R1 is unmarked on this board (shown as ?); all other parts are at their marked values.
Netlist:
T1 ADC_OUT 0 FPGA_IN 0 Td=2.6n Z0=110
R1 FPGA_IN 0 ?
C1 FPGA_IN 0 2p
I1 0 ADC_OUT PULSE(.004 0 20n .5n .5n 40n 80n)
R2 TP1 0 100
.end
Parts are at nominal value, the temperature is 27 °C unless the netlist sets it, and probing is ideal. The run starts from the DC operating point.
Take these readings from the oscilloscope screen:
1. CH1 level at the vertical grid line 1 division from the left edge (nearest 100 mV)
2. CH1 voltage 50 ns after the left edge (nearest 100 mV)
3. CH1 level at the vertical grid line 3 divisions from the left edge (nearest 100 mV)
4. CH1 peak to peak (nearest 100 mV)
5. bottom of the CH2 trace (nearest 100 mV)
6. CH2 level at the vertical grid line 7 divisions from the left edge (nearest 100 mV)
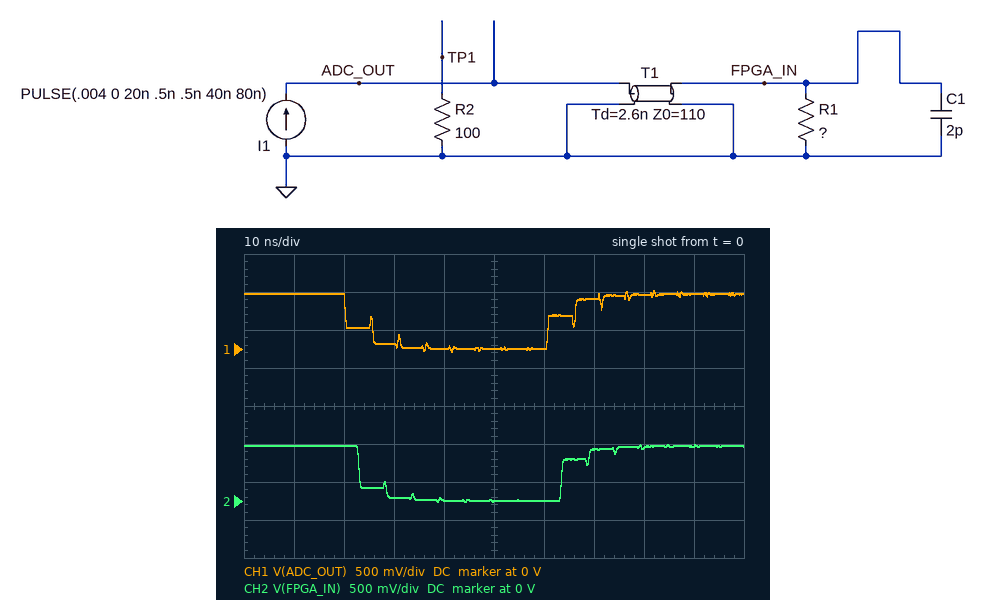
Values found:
700 mV
0 V
100 mV
800 mV
0 V
700 mV
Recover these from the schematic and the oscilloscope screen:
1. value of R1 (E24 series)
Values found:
180 Ω
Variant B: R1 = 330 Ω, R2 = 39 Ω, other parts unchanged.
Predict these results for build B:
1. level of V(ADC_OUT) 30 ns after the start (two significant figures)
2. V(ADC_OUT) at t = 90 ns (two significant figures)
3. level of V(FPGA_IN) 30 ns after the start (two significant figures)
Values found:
440 mV
1.3 V
330 mV
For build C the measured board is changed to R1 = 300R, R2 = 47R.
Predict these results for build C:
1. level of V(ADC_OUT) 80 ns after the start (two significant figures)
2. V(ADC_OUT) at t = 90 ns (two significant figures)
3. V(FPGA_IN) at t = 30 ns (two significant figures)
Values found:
1.1 V
1.2 V
260 mV
